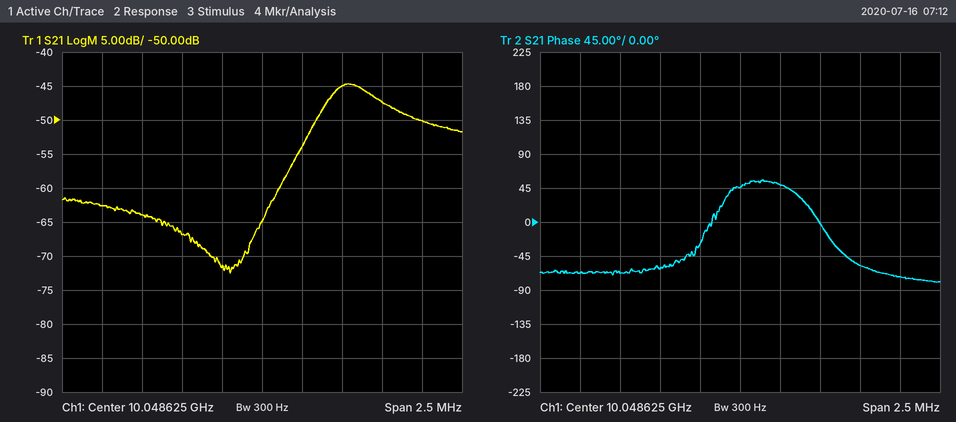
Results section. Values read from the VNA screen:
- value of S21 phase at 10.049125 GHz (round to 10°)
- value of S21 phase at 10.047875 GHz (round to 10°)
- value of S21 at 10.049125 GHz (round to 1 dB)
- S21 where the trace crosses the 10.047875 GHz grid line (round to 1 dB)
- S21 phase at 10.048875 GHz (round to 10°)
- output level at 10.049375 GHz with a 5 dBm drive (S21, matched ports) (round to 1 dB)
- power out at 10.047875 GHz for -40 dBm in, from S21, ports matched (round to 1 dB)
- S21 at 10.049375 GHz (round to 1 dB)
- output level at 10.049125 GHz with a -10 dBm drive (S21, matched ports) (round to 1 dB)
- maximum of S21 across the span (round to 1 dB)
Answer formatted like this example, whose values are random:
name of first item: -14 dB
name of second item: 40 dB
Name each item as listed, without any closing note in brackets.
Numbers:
value of S21 phase at 10.049125 GHz: 0°
value of S21 phase at 10.047875 GHz: -70°
value of S21 at 10.049125 GHz: -45 dB
S21 where the trace crosses the 10.047875 GHz grid line: -64 dB
S21 phase at 10.048875 GHz: 50°
output level at 10.049375 GHz with a 5 dBm drive (S21, matched ports): -42 dBm
power out at 10.047875 GHz for -40 dBm in, from S21, ports matched: -104 dBm
S21 at 10.049375 GHz: -47 dB
output level at 10.049125 GHz with a -10 dBm drive (S21, matched ports): -55 dBm
maximum of S21 across the span: -45 dB
